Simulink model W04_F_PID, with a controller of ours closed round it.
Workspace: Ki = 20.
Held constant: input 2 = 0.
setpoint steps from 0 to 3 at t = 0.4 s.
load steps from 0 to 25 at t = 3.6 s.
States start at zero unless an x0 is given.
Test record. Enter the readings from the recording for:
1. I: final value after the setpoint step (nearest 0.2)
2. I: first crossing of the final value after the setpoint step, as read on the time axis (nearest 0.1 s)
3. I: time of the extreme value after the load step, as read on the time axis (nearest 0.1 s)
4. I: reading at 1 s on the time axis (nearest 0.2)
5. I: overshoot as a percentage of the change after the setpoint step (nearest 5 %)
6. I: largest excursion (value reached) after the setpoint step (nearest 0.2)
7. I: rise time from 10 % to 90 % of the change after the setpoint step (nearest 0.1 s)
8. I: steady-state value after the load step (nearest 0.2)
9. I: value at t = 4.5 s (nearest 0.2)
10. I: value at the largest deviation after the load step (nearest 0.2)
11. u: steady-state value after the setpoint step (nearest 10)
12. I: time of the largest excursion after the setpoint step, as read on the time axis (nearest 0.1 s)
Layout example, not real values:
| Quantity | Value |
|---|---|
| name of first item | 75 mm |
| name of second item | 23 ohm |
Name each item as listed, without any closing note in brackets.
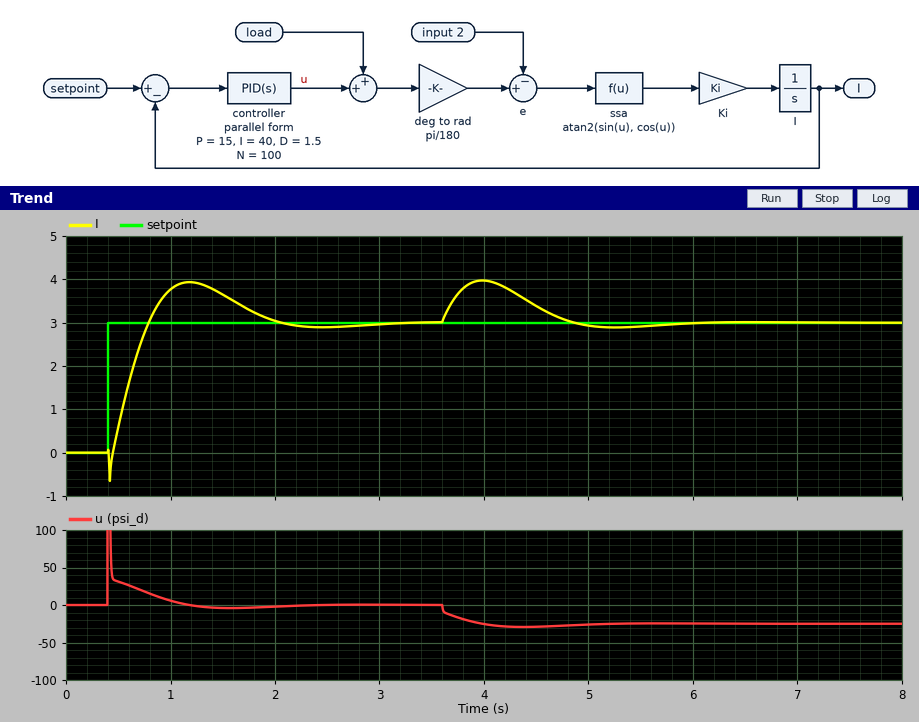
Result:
| Quantity | Value |
|---|---|
| I: final value after the setpoint step | 3.0 |
| I: first crossing of the final value after the setpoint step, as read on the time axis | 0.8 s |
| I: time of the extreme value after the load step, as read on the time axis | 4.0 s |
| I: reading at 1 s on the time axis | 3.8 |
| I: overshoot as a percentage of the change after the setpoint step | 30 % |
| I: largest excursion (value reached) after the setpoint step | 4.0 |
| I: rise time from 10 % to 90 % of the change after the setpoint step | 0.3 s |
| I: steady-state value after the load step | 3.0 |
| I: value at t = 4.5 s | 3.4 |
| I: value at the largest deviation after the load step | 4.0 |
| u: steady-state value after the setpoint step | 0 |
| I: time of the largest excursion after the setpoint step, as read on the time axis | 1.2 s |
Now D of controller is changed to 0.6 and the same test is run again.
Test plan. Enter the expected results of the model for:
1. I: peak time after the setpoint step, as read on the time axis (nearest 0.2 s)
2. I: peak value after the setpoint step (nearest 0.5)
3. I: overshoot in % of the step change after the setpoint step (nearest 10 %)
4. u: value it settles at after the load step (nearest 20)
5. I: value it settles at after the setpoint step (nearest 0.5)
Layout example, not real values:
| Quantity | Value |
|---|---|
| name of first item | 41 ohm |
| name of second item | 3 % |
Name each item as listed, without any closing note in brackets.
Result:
| Quantity | Value |
|---|---|
| I: peak time after the setpoint step, as read on the time axis | 1.0 s |
| I: peak value after the setpoint step | 3.5 |
| I: overshoot in % of the step change after the setpoint step | 20 % |
| u: value it settles at after the load step | -20 |
| I: value it settles at after the setpoint step | 3.0 |
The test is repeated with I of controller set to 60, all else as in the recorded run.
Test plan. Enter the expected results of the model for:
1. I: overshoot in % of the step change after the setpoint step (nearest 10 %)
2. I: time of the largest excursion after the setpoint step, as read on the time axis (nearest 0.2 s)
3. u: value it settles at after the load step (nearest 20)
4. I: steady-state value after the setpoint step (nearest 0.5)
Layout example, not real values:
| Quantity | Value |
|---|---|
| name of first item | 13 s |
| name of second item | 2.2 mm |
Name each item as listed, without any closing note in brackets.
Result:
| Quantity | Value |
|---|---|
| I: overshoot in % of the step change after the setpoint step | 40 % |
| I: time of the largest excursion after the setpoint step, as read on the time axis | 1.0 s |
| u: value it settles at after the load step | -20 |
| I: steady-state value after the setpoint step | 3.0 |
